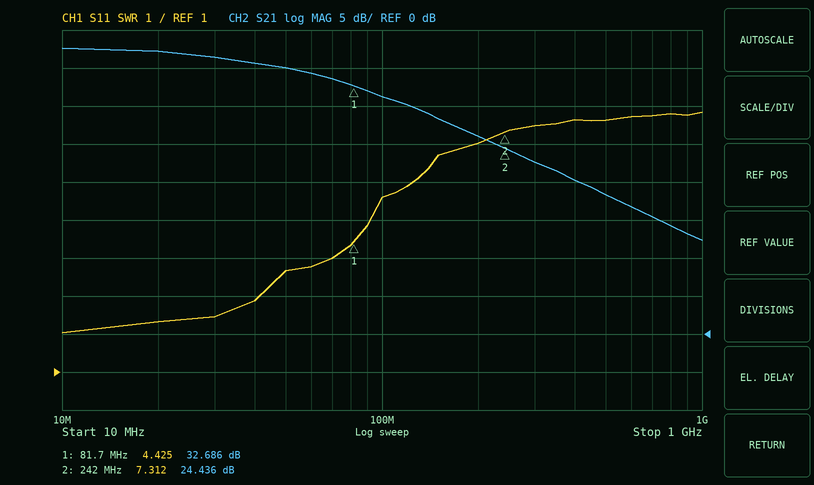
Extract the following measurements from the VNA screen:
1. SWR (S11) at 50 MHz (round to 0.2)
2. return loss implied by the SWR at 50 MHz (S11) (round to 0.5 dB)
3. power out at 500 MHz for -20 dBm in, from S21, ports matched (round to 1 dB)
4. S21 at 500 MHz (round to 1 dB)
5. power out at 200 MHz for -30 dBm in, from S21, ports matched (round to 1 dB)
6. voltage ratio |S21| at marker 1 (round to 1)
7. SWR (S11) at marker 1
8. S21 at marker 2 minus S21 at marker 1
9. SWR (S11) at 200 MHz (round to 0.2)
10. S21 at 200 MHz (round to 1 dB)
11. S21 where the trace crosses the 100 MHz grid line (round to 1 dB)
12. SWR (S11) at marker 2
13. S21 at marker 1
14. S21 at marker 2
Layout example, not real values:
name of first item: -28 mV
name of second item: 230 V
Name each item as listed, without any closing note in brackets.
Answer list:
SWR (S11) at 50 MHz: 3.6
return loss implied by the SWR at 50 MHz (S11): 5.0 dB
power out at 500 MHz for -20 dBm in, from S21, ports matched: -2 dBm
S21 at 500 MHz: 18 dB
power out at 200 MHz for -30 dBm in, from S21, ports matched: -4 dBm
voltage ratio |S21| at marker 1: 43
SWR (S11) at marker 1: 4.425
S21 at marker 2 minus S21 at marker 1: -8.250 dB
SWR (S11) at 200 MHz: 7.0
S21 at 200 MHz: 26 dB
S21 where the trace crosses the 100 MHz grid line: 31 dB
SWR (S11) at marker 2: 7.312
S21 at marker 1: 32.686 dB
S21 at marker 2: 24.436 dB
